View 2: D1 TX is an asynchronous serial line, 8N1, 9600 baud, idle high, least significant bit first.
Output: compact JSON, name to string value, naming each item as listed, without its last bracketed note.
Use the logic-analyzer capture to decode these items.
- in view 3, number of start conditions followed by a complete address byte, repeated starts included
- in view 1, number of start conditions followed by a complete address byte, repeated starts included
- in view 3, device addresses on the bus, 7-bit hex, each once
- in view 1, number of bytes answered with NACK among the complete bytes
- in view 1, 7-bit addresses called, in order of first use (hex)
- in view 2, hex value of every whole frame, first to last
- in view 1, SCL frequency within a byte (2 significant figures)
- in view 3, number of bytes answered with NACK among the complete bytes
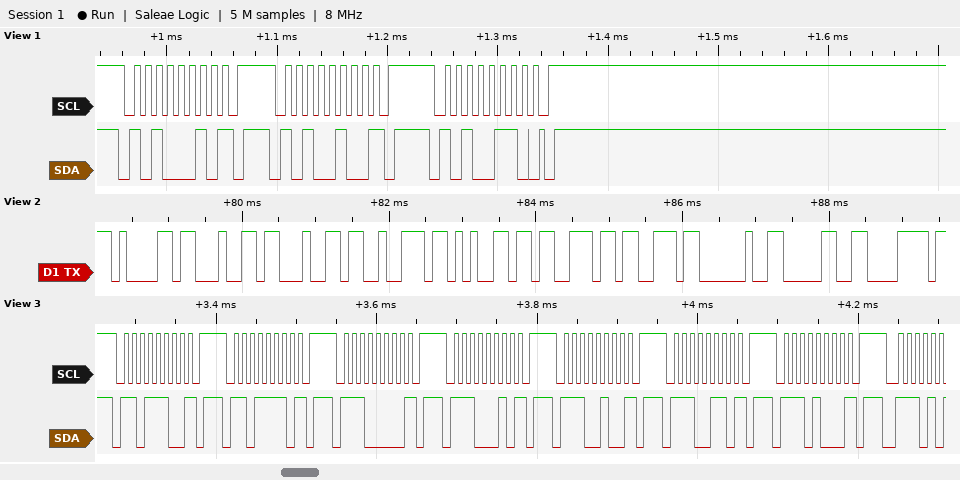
{"in view 3, number of start conditions followed by a complete address byte, repeated starts included": "7", "in view 1, number of start conditions followed by a complete address byte, repeated starts included": "3", "in view 3, device addresses on the bus, 7-bit hex, each once": "0x6E 0x6F 0x70 0x71 0x72 0x73 0x74", "in view 1, number of bytes answered with NACK among the complete bytes": "2", "in view 1, 7-bit addresses called, in order of first use": "0x51 0x52 0x53", "in view 2, hex value of every whole frame, first to last": "61 64 64 72 65 73 73 20 30 78", "in view 1, SCL frequency within a byte": "100 kHz", "in view 3, number of bytes answered with NACK among the complete bytes": "7"}
